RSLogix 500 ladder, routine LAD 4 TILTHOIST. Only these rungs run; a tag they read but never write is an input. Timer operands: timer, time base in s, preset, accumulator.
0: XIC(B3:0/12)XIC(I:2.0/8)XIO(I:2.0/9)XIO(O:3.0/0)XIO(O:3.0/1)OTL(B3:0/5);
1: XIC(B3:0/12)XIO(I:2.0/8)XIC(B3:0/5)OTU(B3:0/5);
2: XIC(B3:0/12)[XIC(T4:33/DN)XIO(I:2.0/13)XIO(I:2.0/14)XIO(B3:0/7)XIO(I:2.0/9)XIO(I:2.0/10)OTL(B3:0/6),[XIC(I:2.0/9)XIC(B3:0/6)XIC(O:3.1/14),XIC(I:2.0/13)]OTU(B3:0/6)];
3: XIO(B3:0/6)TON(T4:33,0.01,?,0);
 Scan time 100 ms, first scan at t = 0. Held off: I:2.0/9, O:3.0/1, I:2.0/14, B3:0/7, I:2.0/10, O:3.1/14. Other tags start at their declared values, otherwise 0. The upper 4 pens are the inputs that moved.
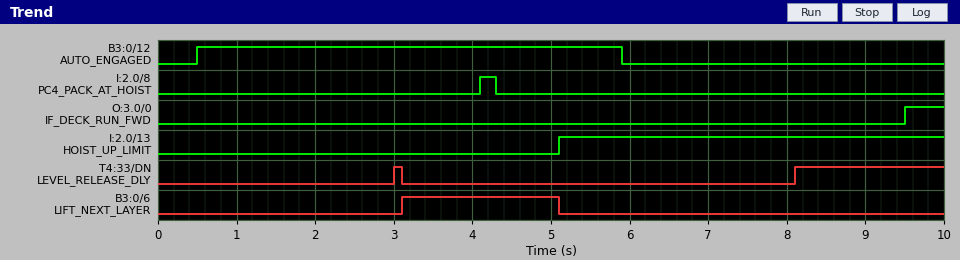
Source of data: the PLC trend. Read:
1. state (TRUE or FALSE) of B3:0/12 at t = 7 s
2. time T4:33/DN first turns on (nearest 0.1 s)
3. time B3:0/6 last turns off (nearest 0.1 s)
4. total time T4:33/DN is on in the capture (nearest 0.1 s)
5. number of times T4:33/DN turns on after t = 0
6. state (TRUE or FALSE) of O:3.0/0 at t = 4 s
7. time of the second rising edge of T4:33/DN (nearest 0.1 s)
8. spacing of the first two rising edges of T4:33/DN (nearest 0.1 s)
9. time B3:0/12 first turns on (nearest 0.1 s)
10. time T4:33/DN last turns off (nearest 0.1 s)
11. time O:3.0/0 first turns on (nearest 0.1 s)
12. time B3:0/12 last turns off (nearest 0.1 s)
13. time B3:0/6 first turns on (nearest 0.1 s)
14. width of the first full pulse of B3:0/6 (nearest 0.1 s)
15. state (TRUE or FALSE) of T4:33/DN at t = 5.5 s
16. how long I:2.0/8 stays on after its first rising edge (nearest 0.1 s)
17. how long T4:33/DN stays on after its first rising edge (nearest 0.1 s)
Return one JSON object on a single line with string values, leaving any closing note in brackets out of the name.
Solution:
{"state (TRUE or FALSE) of B3:0/12 at t = 7 s": "FALSE", "time T4:33/DN first turns on": "3.0 s", "time B3:0/6 last turns off": "5.1 s", "total time T4:33/DN is on in the capture": "2.0 s", "number of times T4:33/DN turns on after t = 0": "2", "state (TRUE or FALSE) of O:3.0/0 at t = 4 s": "FALSE", "time of the second rising edge of T4:33/DN": "8.1 s", "spacing of the first two rising edges of T4:33/DN": "5.1 s", "time B3:0/12 first turns on": "0.5 s", "time T4:33/DN last turns off": "3.1 s", "time O:3.0/0 first turns on": "9.5 s", "time B3:0/12 last turns off": "5.9 s", "time B3:0/6 first turns on": "3.1 s", "width of the first full pulse of B3:0/6": "2.0 s", "state (TRUE or FALSE) of T4:33/DN at t = 5.5 s": "FALSE", "how long I:2.0/8 stays on after its first rising edge": "0.2 s", "how long T4:33/DN stays on after its first rising edge": "0.1 s"}
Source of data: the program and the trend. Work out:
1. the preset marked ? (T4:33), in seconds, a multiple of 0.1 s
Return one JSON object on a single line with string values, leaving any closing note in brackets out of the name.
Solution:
{"the preset marked ? (T4:33), in seconds, a multiple of 0.1 s": "3.0 s"}
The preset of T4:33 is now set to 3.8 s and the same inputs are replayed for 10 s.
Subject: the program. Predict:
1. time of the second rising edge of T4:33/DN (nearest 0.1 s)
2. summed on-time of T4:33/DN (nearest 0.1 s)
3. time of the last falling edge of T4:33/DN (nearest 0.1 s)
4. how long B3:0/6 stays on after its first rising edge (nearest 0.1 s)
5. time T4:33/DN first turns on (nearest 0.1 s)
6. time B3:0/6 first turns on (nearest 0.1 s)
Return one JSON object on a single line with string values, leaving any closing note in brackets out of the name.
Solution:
{"time of the second rising edge of T4:33/DN": "8.9 s", "summed on-time of T4:33/DN": "1.2 s", "time of the last falling edge of T4:33/DN": "3.9 s", "how long B3:0/6 stays on after its first rising edge": "1.2 s", "time T4:33/DN first turns on": "3.8 s", "time B3:0/6 first turns on": "3.9 s"}
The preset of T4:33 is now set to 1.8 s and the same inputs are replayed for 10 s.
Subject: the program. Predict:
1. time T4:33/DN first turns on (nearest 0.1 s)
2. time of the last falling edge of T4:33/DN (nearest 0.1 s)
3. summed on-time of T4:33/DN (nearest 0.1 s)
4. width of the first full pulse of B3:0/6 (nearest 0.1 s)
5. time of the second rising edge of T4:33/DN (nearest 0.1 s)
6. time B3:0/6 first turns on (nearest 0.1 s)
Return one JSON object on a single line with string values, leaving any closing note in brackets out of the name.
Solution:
{"time T4:33/DN first turns on": "1.8 s", "time of the last falling edge of T4:33/DN": "1.9 s", "summed on-time of T4:33/DN": "3.2 s", "width of the first full pulse of B3:0/6": "3.2 s", "time of the second rising edge of T4:33/DN": "6.9 s", "time B3:0/6 first turns on": "1.9 s"}
